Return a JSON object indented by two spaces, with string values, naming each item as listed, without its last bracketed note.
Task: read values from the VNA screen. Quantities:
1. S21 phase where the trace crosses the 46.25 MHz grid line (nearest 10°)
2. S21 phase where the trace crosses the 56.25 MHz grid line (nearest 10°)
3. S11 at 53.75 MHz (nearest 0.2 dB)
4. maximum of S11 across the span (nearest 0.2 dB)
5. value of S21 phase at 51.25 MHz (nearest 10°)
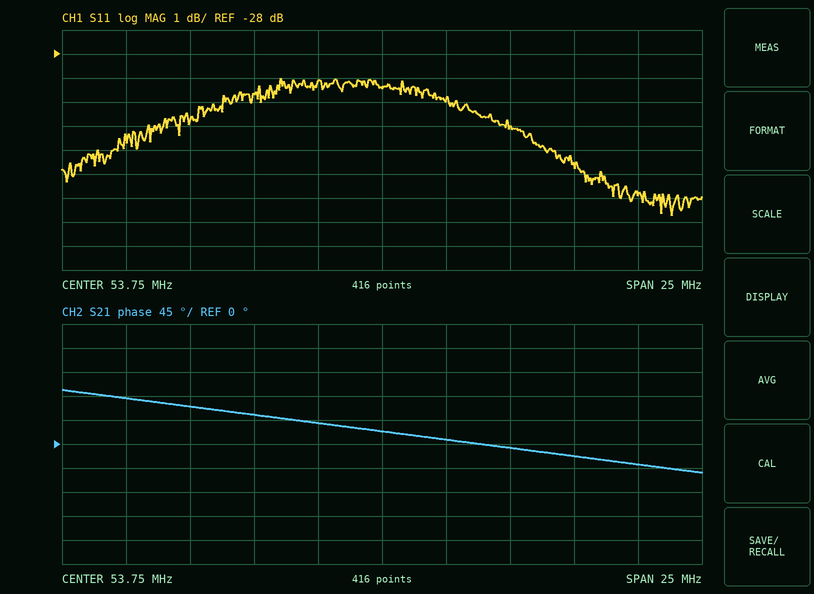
{
  "S21 phase where the trace crosses the 46.25 MHz grid line": "70°",
  "S21 phase where the trace crosses the 56.25 MHz grid line": "10°",
  "S11 at 53.75 MHz": "-29.4 dB",
  "maximum of S11 across the span": "-29.0 dB",
  "value of S21 phase at 51.25 MHz": "40°"
}
